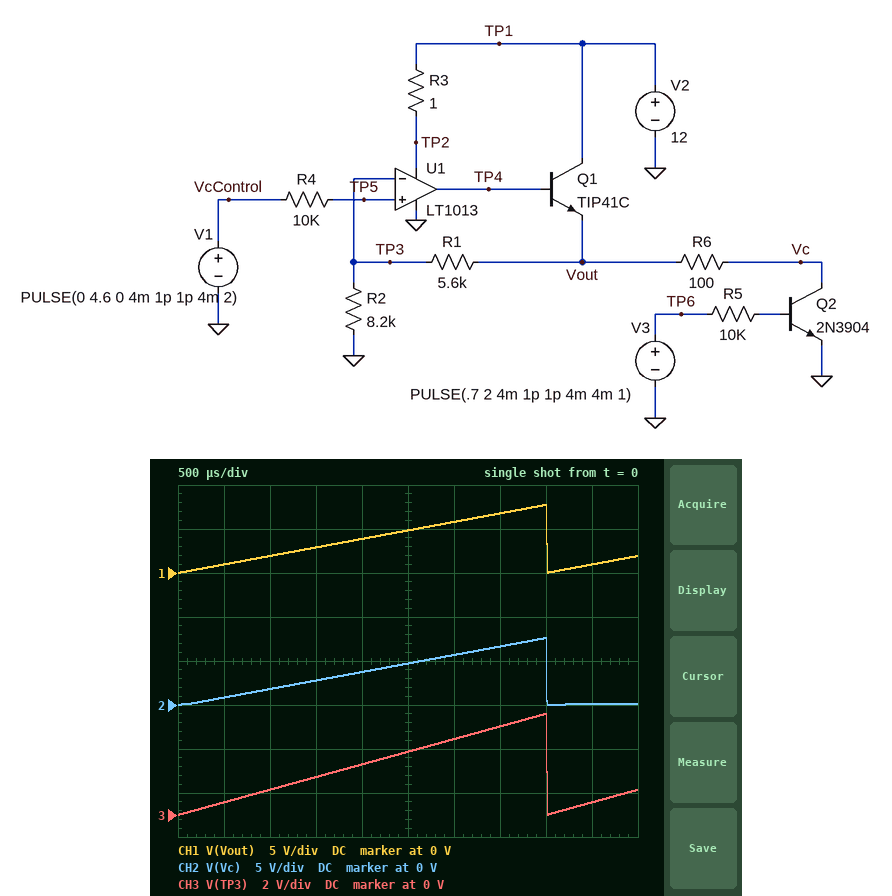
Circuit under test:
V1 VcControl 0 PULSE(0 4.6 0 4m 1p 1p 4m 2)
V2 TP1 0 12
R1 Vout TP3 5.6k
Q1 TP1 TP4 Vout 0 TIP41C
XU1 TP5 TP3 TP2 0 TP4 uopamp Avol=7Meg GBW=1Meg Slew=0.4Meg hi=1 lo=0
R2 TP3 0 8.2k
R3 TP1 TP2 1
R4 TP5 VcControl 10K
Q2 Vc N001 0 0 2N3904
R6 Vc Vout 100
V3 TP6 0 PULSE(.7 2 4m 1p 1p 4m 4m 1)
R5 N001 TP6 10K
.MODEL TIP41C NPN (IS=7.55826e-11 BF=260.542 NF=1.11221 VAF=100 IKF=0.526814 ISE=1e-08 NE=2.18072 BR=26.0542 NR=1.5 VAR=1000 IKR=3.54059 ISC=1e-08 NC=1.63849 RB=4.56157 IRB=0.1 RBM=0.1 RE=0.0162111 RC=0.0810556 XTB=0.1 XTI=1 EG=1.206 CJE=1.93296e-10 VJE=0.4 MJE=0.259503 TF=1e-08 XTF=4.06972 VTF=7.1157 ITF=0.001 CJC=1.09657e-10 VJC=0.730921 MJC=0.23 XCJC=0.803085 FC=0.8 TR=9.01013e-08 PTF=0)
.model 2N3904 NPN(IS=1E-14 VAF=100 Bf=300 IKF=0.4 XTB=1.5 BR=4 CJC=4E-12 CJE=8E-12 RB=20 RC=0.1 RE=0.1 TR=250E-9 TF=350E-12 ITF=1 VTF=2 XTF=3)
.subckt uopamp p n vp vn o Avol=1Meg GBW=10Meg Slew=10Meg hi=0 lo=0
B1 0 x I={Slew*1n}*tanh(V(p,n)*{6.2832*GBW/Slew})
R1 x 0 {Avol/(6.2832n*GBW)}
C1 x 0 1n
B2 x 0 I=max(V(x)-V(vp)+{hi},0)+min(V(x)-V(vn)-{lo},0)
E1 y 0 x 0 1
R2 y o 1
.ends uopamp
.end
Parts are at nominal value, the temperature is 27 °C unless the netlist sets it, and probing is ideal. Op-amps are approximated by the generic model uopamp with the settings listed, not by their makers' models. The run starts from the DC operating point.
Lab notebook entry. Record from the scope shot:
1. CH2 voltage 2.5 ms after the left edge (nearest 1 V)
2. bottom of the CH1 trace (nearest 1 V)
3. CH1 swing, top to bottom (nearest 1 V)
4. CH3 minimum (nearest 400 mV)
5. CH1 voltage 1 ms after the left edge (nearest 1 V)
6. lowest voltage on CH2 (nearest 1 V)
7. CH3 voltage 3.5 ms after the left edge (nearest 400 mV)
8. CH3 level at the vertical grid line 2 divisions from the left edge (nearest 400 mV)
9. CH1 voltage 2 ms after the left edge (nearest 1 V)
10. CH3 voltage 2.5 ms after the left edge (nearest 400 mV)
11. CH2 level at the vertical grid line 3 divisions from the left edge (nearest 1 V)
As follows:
5 V
0 V
8 V
0 V
2 V
0 V
4.0 V
1.2 V
4 V
2.8 V
3 V
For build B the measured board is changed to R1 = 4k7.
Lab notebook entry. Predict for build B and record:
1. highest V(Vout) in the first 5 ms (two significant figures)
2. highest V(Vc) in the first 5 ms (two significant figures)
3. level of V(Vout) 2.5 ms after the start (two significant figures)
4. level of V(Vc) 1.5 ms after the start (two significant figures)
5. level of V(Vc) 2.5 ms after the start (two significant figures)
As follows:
7.2 V
7.1 V
4.5 V
2.6 V
4.4 V
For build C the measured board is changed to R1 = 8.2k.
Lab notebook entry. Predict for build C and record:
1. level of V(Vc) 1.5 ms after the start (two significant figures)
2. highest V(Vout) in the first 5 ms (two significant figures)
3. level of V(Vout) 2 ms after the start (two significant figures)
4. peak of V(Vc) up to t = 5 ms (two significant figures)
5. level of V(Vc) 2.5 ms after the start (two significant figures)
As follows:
3.3 V
9.2 V
4.6 V
9.1 V
5.6 V
